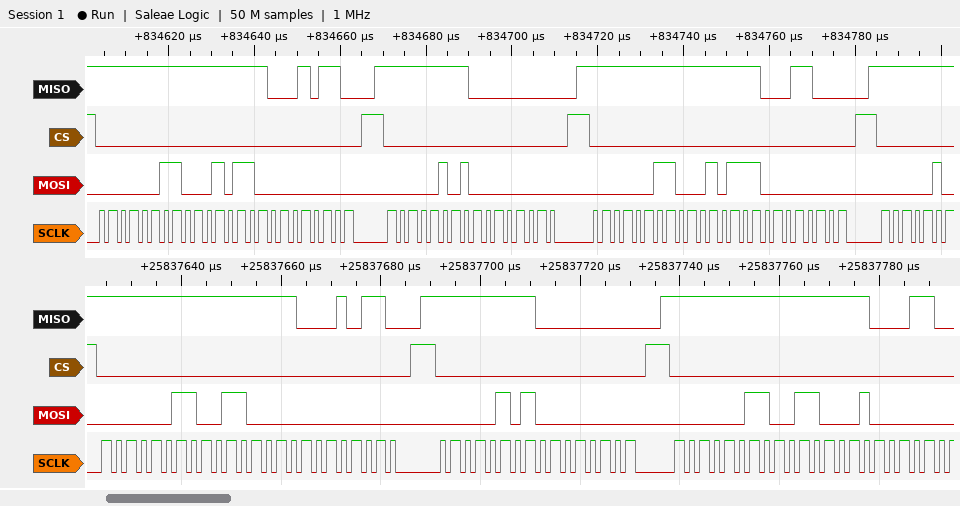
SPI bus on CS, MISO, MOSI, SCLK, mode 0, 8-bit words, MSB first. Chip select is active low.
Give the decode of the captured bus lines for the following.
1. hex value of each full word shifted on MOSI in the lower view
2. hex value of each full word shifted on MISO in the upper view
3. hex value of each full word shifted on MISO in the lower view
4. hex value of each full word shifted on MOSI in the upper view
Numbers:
03, 30, 00, 05, 00, 03, 31
FF, FF, 16, FF, 00, FF, FF, 18
FF, FF, 16, FF, 00, FF, FF
03, 16, 00, 05, 00, 03, 17, 00
